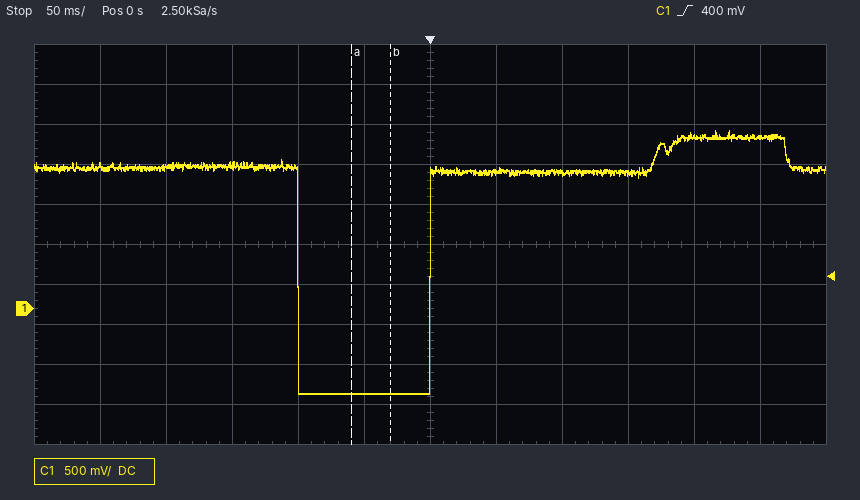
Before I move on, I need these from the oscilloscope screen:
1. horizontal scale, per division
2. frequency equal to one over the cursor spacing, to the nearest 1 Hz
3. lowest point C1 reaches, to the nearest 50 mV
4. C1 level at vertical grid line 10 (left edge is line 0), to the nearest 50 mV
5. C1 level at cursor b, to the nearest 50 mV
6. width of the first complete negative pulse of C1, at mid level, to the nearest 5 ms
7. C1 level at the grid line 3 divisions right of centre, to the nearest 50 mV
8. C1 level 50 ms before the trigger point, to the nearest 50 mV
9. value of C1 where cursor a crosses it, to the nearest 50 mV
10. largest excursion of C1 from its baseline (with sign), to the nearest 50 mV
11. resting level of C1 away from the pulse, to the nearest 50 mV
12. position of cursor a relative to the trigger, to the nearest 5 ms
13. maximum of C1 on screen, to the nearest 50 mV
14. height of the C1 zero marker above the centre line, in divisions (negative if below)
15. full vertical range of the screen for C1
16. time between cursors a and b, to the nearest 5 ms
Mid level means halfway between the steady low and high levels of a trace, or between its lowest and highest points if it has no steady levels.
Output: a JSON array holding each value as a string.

["50 ms", "33 Hz", "-1.05 V", "2.15 V", "-1.05 V", "100 ms", "1.70 V", "-1.05 V", "-1.05 V", "-2.80 V", "1.75 V", "-60 ms", "2.20 V", "-1.6 div", "5 V", "30 ms"]
